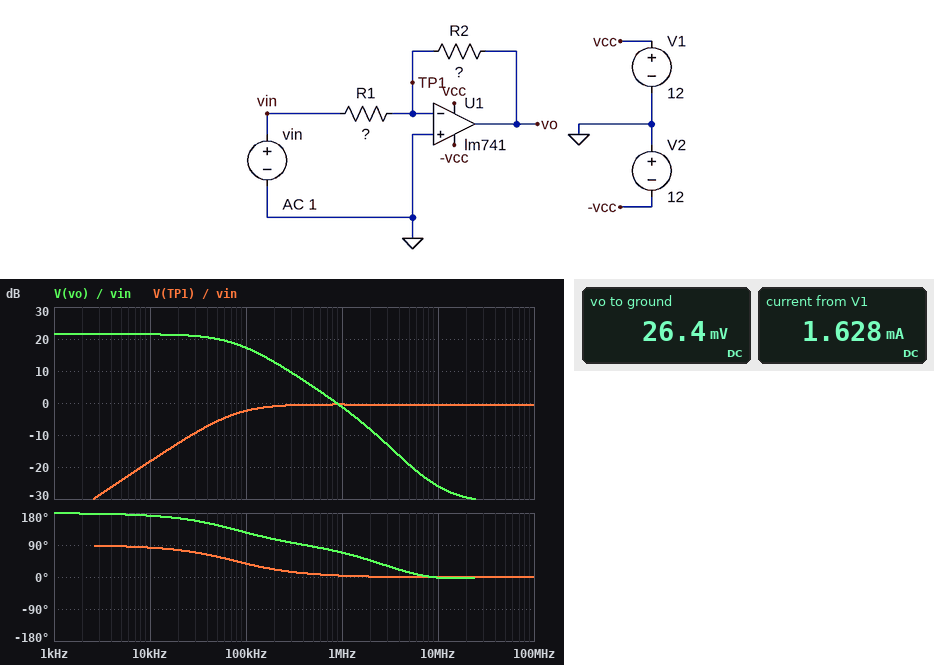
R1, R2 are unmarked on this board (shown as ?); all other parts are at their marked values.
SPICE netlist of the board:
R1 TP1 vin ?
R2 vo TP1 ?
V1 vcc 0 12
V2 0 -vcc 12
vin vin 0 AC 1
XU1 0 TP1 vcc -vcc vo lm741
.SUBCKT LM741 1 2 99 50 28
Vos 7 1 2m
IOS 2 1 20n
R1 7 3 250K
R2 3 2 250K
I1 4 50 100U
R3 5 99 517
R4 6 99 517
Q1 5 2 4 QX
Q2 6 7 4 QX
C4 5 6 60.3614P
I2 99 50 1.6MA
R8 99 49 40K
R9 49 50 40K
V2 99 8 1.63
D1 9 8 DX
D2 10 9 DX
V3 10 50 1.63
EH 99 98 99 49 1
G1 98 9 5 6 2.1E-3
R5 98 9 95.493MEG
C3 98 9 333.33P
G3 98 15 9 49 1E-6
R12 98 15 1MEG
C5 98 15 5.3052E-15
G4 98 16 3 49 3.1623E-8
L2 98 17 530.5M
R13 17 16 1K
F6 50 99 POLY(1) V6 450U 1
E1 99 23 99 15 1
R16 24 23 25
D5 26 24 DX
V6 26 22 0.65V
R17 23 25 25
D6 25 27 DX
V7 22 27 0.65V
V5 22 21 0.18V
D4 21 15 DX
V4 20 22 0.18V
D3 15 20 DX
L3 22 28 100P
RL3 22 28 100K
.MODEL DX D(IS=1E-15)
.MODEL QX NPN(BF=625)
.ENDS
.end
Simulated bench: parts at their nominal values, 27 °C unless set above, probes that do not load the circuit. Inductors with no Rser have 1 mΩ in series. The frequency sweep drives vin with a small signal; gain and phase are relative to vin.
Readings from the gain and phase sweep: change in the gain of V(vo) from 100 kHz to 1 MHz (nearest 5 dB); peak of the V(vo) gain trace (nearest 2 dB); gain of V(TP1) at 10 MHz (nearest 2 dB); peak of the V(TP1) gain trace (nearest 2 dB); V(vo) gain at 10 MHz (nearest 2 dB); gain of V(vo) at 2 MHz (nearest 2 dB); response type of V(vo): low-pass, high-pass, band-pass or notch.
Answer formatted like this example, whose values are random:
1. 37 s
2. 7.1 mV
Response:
1. -20 dB
2. 22 dB
3. 0 dB
4. 0 dB
5. -26 dB
6. -8 dB
7. low-pass
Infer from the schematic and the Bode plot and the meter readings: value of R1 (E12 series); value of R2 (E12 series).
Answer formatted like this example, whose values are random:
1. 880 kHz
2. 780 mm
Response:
1. 470 Ω
2. 5.6 kΩ
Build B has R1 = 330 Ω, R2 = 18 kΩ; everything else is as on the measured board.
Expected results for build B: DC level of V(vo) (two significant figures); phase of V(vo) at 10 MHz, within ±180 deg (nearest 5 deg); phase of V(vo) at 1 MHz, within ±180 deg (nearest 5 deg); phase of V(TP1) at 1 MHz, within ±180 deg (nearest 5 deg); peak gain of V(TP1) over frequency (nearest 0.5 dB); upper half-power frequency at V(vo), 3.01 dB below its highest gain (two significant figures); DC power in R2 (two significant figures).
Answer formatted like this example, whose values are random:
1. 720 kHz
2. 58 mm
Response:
1. 110 mV
2. -5 deg
3. 65 deg
4. 0 deg
5. 0 dB
6. 18 kHz
7. 680 nW
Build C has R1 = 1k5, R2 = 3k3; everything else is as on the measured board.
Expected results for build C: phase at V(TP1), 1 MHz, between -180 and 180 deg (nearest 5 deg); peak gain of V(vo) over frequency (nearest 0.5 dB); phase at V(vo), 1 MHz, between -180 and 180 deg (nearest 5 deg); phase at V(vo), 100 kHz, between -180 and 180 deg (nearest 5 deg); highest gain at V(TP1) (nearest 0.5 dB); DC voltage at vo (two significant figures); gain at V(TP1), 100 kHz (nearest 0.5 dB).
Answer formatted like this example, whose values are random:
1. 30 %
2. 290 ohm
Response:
1. 15 deg
2. 7.0 dB
3. 80 deg
4. 160 deg
5. -2.5 dB
6. 6.7 mV
7. -13.0 dB
